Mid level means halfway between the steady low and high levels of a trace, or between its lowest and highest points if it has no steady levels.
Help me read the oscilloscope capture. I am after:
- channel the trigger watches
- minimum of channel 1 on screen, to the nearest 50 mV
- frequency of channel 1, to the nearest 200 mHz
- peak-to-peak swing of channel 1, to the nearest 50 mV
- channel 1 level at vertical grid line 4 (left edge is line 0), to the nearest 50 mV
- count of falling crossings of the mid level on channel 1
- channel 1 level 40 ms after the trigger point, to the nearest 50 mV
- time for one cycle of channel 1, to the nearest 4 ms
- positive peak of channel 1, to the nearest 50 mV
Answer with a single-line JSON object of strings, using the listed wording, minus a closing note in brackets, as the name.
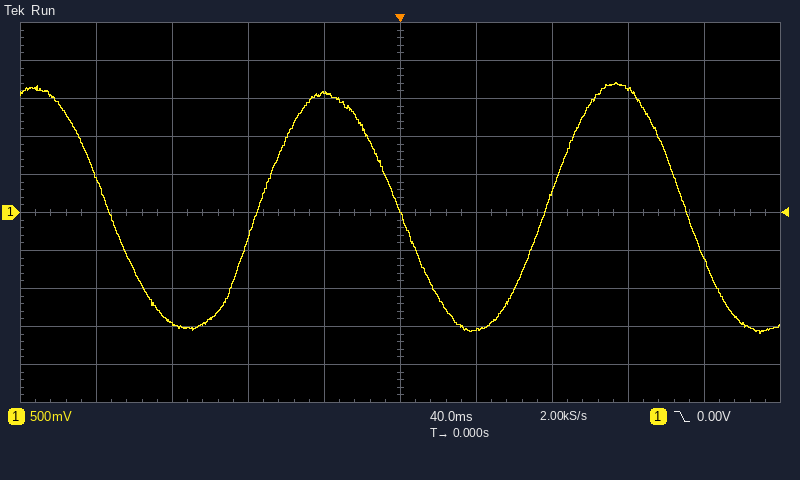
{"channel the trigger watches": "channel 1", "minimum of channel 1 on screen, to the nearest 50 mV": "-1.60 V", "frequency of channel 1, to the nearest 200 mHz": "6.6 Hz", "peak-to-peak swing of channel 1, to the nearest 50 mV": "3.30 V", "channel 1 level at vertical grid line 4 (left edge is line 0), to the nearest 50 mV": "1.55 V", "count of falling crossings of the mid level on channel 1": "3", "channel 1 level 40 ms after the trigger point, to the nearest 50 mV": "-1.55 V", "time for one cycle of channel 1, to the nearest 4 ms": "152 ms", "positive peak of channel 1, to the nearest 50 mV": "1.70 V"}
